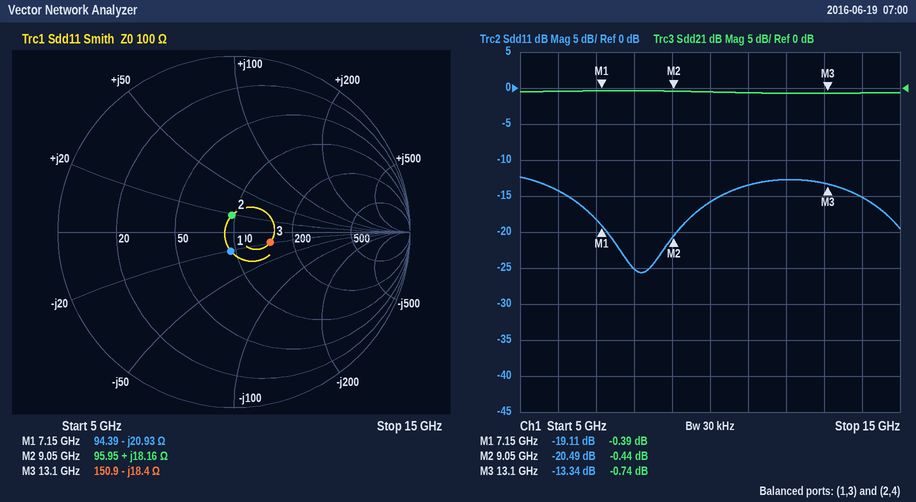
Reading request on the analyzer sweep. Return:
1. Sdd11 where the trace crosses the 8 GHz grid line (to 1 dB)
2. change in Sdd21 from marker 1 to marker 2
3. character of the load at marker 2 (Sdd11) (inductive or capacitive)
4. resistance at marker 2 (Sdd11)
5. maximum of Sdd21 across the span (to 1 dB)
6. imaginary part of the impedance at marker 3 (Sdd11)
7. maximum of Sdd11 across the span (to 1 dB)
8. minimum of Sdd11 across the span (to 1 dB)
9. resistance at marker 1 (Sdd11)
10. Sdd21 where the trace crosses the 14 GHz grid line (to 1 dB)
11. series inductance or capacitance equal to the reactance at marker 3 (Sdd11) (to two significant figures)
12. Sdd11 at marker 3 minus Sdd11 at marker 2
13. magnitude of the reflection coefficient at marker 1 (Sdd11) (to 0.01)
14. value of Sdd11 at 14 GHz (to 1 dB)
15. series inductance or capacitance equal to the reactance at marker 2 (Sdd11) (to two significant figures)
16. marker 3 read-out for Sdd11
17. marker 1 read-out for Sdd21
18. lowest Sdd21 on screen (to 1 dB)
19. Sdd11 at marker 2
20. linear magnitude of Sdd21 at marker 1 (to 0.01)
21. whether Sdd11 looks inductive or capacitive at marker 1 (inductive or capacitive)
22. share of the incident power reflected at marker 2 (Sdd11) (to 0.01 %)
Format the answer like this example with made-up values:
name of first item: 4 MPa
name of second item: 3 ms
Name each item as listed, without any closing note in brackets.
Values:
Sdd11 where the trace crosses the 8 GHz grid line: -25 dB
change in Sdd21 from marker 1 to marker 2: -0.05 dB
character of the load at marker 2 (Sdd11): inductive
resistance at marker 2: 95.95 Ω
maximum of Sdd21 across the span: 0 dB
imaginary part of the impedance at marker 3: -18.4 Ω
maximum of Sdd11 across the span: -12 dB
minimum of Sdd11 across the span: -26 dB
resistance at marker 1: 94.39 Ω
Sdd21 where the trace crosses the 14 GHz grid line: -1 dB
series inductance or capacitance equal to the reactance at marker 3 (Sdd11): 660 fF
Sdd11 at marker 3 minus Sdd11 at marker 2: 7.15 dB
magnitude of the reflection coefficient at marker 1 (Sdd11): 0.11
value of Sdd11 at 14 GHz: -15 dB
series inductance or capacitance equal to the reactance at marker 2 (Sdd11): 320 pH
marker 3 read-out for Sdd11: -13.34 dB
marker 1 read-out for Sdd21: -0.39 dB
lowest Sdd21 on screen: -1 dB
Sdd11 at marker 2: -20.49 dB
linear magnitude of Sdd21 at marker 1: 0.96
whether Sdd11 looks inductive or capacitive at marker 1: capacitive
share of the incident power reflected at marker 2 (Sdd11): 0.89 %
